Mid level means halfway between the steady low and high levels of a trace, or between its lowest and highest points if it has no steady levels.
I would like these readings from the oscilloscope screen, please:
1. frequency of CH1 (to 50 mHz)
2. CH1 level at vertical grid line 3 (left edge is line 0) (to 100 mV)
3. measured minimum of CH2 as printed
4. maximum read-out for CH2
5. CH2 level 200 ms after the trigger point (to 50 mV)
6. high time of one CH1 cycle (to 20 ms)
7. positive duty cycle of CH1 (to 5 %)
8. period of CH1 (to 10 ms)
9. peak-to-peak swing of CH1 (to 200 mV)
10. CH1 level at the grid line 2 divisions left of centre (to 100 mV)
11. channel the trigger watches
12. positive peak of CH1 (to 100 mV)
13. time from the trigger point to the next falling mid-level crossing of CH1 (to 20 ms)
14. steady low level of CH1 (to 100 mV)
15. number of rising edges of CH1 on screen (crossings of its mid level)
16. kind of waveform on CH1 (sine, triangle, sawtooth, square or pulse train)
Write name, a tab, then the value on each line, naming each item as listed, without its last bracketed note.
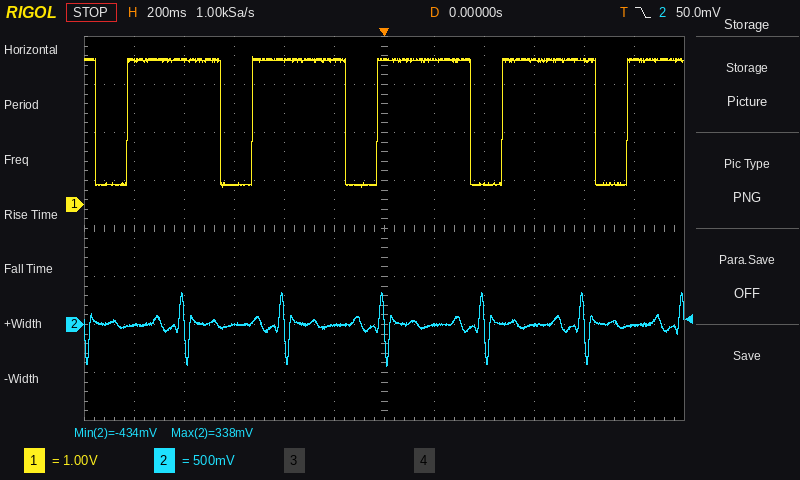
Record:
frequency of CH1	2.00 Hz
CH1 level at vertical grid line 3 (left edge is line 0)	400 mV
measured minimum of CH2 as printed	-434 mV
maximum read-out for CH2	338 mV
CH2 level 200 ms after the trigger point	0 mV
high time of one CH1 cycle	380 ms
positive duty cycle of CH1	75 %
period of CH1	500 ms
peak-to-peak swing of CH1	2.8 V
CH1 level at the grid line 2 divisions left of centre	3.0 V
channel the trigger watches	CH2
positive peak of CH1	3.1 V
time from the trigger point to the next falling mid-level crossing of CH1	340 ms
steady low level of CH1	400 mV
number of rising edges of CH1 on screen	5
kind of waveform on CH1	pulse train
